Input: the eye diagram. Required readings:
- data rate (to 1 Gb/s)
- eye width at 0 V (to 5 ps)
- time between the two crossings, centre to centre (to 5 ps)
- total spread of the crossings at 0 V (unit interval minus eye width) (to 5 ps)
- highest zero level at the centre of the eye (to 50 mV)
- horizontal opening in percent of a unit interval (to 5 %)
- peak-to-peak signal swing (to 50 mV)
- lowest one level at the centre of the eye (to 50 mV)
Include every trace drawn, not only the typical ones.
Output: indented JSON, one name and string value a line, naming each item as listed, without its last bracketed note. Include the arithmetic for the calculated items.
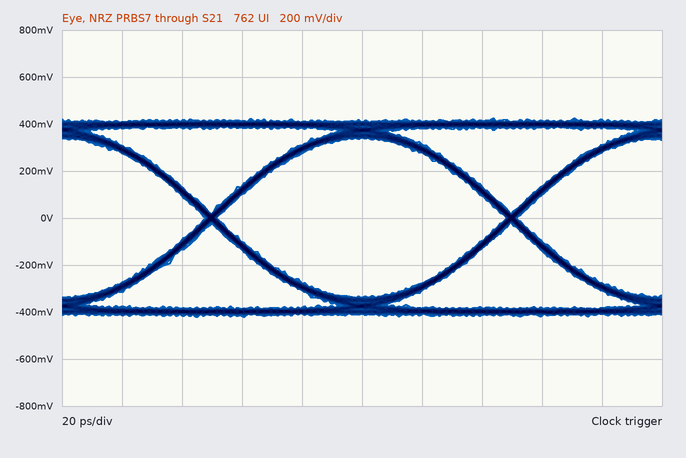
{
  "data rate": "10 Gb/s",
  "eye width at 0 V": "95 ps",
  "time between the two crossings, centre to centre": "100 ps",
  "total spread of the crossings at 0 V (unit interval minus eye width)": "5 ps",
  "highest zero level at the centre of the eye": "-350 mV",
  "horizontal opening in percent of a unit interval": "95 ps / 100 ps ≈ 95 %",
  "peak-to-peak signal swing": "850 mV",
  "lowest one level at the centre of the eye": "350 mV"
}
